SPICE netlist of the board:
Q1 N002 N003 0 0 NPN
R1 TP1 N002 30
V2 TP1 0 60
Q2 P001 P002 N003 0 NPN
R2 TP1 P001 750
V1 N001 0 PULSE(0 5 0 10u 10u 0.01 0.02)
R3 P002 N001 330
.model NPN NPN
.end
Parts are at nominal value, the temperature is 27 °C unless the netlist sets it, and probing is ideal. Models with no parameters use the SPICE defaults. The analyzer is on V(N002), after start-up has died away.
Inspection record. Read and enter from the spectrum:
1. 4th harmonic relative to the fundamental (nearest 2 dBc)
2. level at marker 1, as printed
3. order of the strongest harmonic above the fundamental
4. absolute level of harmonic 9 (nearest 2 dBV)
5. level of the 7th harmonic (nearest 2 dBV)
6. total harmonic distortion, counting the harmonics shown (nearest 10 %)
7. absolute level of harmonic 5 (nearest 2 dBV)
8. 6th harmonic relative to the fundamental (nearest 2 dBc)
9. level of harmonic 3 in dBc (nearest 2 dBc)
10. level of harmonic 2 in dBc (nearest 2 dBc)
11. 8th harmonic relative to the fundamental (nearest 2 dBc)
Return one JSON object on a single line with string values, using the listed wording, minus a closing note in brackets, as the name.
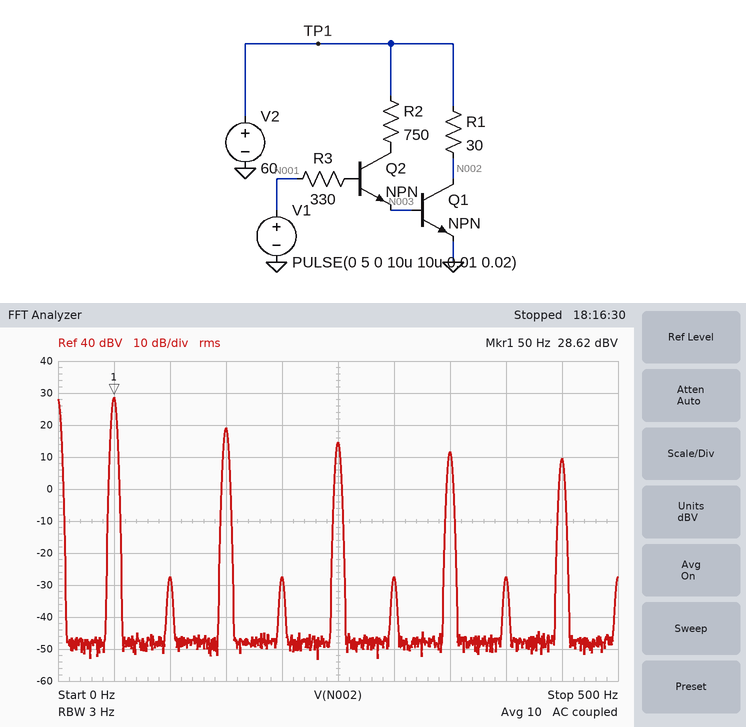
{"4th harmonic relative to the fundamental": "-56 dBc", "level at marker 1, as printed": "28.62 dBV", "order of the strongest harmonic above the fundamental": "3", "absolute level of harmonic 9": "10 dBV", "level of the 7th harmonic": "12 dBV", "total harmonic distortion, counting the harmonics shown": "40 %", "absolute level of harmonic 5": "14 dBV", "6th harmonic relative to the fundamental": "-56 dBc", "level of harmonic 3 in dBc": "-10 dBc", "level of harmonic 2 in dBc": "-56 dBc", "8th harmonic relative to the fundamental": "-56 dBc"}
